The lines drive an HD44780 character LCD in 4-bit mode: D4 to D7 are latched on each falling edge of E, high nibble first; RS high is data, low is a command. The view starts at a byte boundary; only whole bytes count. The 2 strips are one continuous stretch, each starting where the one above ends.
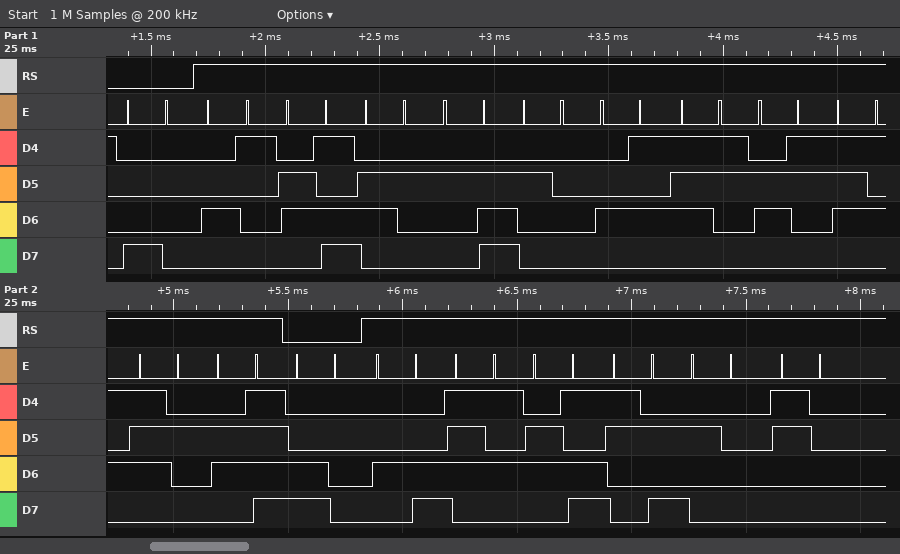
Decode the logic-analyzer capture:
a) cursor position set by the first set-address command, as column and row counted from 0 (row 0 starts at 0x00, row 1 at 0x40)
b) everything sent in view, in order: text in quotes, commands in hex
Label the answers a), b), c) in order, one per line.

a) column 0, row 0
b) 0x80 "Amb. Escuro" 0xC0 "Lum: 0"
